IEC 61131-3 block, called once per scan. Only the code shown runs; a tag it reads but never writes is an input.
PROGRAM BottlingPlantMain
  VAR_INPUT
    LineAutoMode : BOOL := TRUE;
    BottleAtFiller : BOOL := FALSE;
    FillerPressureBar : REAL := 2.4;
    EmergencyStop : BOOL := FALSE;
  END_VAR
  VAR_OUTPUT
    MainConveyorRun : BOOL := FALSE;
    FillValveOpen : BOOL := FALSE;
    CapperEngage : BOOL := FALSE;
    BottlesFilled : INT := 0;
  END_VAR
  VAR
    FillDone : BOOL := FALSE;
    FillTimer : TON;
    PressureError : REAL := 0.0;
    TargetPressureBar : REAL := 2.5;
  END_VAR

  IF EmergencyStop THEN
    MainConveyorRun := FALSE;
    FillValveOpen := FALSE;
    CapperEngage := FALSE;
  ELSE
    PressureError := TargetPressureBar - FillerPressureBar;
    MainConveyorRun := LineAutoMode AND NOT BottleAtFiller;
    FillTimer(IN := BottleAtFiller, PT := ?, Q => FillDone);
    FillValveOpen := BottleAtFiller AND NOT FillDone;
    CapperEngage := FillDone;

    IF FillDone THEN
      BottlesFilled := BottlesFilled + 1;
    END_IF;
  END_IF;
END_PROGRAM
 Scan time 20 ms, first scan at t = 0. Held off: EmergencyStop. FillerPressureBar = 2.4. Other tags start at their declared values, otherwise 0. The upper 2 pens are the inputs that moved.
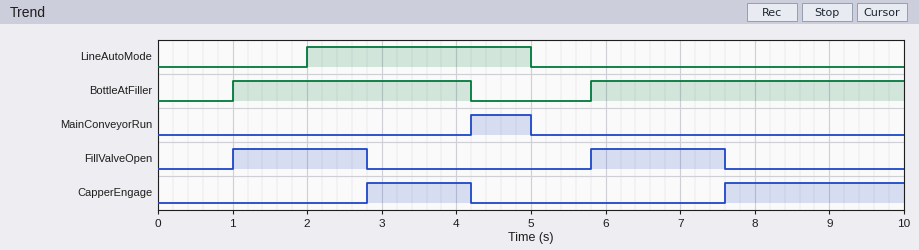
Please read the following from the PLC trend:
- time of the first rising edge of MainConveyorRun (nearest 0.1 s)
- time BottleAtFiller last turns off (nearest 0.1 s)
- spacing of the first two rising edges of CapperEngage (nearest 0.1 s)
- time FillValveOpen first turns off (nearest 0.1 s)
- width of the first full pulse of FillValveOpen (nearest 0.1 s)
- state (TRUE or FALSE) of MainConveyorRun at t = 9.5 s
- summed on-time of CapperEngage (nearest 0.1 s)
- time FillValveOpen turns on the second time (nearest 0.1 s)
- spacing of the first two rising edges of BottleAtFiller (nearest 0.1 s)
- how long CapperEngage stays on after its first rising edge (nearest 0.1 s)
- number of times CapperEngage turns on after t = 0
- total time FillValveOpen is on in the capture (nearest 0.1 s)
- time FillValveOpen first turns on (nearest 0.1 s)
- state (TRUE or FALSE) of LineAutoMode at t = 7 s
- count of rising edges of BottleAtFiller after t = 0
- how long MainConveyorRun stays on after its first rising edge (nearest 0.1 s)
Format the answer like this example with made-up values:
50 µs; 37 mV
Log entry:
4.2 s; 4.2 s; 4.8 s; 2.8 s; 1.8 s; FALSE; 3.8 s; 5.8 s; 4.8 s; 1.4 s; 2; 3.6 s; 1.0 s; FALSE; 2; 0.8 s
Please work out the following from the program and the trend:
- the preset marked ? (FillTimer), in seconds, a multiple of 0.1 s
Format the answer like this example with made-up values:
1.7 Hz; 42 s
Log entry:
1.8 s
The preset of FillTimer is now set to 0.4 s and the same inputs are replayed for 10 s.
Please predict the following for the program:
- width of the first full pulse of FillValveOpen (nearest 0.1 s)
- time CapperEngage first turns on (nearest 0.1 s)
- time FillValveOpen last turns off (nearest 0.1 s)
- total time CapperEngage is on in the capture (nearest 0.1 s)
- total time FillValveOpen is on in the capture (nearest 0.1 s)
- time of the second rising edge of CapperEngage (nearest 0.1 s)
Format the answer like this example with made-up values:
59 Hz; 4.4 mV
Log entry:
0.4 s; 1.4 s; 6.2 s; 6.6 s; 0.8 s; 6.2 s
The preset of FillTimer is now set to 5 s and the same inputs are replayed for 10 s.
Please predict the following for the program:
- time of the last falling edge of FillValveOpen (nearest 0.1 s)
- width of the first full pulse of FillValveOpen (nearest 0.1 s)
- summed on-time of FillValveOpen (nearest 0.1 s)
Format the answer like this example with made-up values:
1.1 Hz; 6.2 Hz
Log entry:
4.2 s; 3.2 s; 7.4 s
